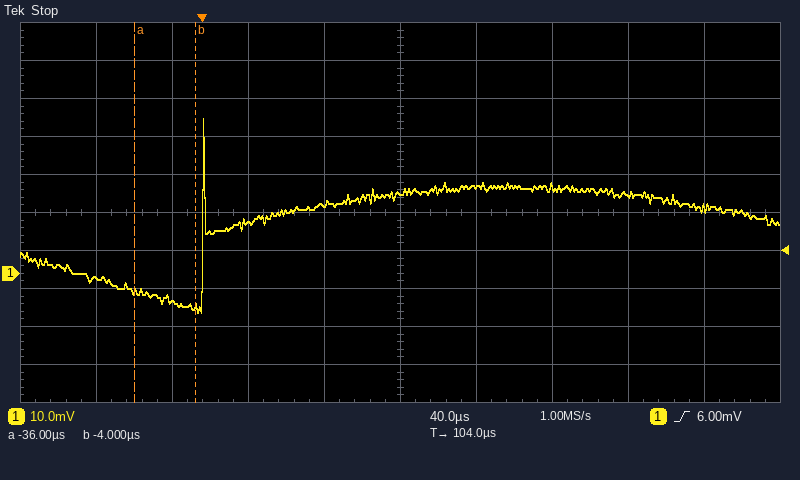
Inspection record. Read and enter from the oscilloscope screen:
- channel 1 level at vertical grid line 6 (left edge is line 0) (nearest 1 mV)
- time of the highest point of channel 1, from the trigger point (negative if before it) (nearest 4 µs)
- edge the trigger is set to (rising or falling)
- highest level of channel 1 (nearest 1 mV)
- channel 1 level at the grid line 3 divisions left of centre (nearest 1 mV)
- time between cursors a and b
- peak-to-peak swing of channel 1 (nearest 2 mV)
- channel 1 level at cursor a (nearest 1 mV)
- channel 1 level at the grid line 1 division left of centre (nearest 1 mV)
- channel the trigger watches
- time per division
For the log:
23 mV
0 µs
rising
41 mV
-7 mV
32 µs
52 mV
-5 mV
18 mV
channel 1
40 µs
